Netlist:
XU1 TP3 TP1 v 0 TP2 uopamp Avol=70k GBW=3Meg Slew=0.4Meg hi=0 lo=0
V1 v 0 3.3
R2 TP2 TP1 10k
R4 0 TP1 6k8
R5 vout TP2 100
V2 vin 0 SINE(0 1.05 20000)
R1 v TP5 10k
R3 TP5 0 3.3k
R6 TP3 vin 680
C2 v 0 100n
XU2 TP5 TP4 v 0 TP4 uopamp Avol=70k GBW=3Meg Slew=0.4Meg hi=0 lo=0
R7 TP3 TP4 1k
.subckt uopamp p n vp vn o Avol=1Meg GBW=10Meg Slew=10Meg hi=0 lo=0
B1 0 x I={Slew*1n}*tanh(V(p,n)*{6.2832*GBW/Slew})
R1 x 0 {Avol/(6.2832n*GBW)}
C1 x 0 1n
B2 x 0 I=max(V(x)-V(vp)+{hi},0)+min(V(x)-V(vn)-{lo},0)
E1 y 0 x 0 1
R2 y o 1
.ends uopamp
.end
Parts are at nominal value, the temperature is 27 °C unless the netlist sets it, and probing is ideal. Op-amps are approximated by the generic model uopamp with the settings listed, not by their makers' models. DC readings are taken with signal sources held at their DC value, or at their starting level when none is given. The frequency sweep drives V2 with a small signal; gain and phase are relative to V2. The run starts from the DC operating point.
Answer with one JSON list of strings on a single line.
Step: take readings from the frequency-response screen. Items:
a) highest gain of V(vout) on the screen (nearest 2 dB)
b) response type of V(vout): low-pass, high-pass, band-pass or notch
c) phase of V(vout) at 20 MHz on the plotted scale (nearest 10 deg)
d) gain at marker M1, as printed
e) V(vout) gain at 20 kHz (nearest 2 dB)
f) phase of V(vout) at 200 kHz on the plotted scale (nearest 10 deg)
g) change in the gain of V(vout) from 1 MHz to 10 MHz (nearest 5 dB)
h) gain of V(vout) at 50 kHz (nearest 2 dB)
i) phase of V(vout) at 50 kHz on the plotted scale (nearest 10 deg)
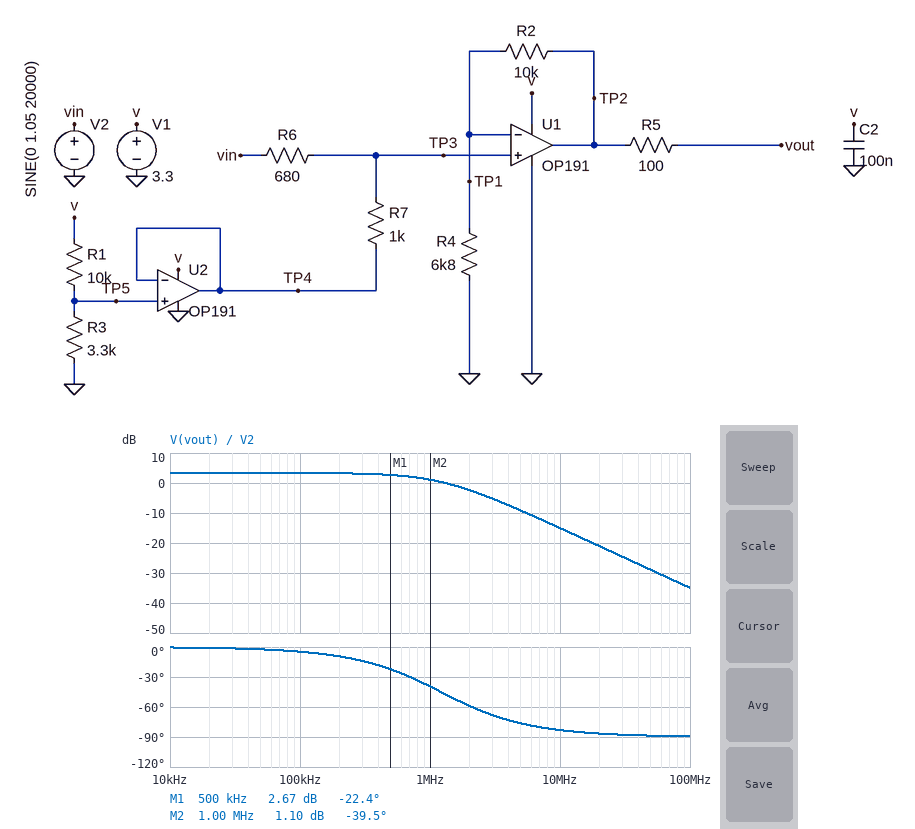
["4 dB", "low-pass", "-90 deg", "2.67 dB", "4 dB", "-10 deg", "-15 dB", "4 dB", "0 deg"]
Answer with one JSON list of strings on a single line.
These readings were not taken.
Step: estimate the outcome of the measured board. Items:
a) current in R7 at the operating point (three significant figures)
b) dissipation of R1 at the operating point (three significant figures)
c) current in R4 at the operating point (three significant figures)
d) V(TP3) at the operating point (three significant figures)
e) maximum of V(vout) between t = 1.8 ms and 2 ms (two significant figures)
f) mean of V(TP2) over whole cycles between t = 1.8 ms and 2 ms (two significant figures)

["487 µA", "616 µW", "48.7 µA", "331 mV", "2.4 V", "970 mV"]
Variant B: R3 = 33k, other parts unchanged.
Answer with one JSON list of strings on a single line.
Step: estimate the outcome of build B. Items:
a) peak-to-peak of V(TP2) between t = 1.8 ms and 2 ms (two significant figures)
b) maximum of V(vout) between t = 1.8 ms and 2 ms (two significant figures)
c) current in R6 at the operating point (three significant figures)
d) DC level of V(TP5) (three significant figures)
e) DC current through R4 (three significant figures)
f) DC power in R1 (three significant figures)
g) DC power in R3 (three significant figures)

["2.3 V", "3.3 V", "1.51 mA", "2.53 V", "151 µA", "58.9 µW", "194 µW"]
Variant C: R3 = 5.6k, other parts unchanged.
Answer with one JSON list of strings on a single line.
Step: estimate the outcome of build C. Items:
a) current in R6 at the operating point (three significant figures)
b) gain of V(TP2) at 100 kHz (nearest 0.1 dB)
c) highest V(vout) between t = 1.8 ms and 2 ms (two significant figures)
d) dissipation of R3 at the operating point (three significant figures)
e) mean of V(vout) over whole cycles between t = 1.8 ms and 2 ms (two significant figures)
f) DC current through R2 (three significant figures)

["705 µA", "3.3 dB", "2.7 V", "251 µW", "1.2 V", "70.5 µA"]
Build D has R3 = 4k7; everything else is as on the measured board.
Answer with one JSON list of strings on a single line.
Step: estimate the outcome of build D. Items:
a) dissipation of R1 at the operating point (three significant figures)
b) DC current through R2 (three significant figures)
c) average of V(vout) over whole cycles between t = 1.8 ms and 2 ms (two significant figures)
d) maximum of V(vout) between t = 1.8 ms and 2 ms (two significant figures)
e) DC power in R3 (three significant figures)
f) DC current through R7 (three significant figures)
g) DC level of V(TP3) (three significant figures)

["504 µW", "62.8 µA", "1.1 V", "2.6 V", "237 µW", "628 µA", "427 mV"]
